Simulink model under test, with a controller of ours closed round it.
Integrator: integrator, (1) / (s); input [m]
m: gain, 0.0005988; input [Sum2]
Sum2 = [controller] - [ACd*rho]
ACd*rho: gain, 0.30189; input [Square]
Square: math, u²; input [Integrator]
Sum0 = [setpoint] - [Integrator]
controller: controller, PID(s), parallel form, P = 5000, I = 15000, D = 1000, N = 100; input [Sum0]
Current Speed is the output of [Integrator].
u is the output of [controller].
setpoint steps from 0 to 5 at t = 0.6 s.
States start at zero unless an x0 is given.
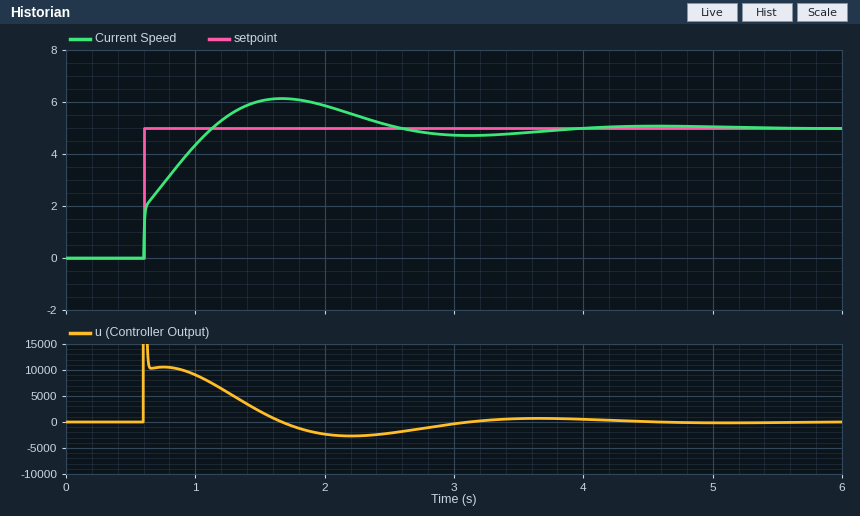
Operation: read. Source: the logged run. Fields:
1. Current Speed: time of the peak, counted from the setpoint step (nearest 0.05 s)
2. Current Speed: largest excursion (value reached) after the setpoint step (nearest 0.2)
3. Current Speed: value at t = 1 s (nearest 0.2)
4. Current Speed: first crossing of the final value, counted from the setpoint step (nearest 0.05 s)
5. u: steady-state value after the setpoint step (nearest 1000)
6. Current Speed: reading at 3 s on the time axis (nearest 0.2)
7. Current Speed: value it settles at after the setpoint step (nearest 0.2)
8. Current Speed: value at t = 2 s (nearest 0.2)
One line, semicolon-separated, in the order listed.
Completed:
1.05 s; 6.2; 4.4; 0.55 s; 0; 4.8; 5.0; 5.8
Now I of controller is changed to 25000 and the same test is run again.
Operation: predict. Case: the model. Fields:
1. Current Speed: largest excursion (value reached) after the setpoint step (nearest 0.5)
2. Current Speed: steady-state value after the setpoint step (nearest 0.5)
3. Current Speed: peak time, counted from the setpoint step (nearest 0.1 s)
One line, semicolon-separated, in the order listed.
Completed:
6.5; 5.0; 0.9 s
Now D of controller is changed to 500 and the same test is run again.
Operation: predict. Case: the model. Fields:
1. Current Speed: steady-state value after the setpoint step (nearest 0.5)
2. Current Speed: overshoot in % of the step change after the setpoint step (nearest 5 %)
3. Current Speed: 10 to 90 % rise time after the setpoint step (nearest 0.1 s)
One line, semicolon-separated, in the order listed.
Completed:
5.0; 25 %; 0.4 s
